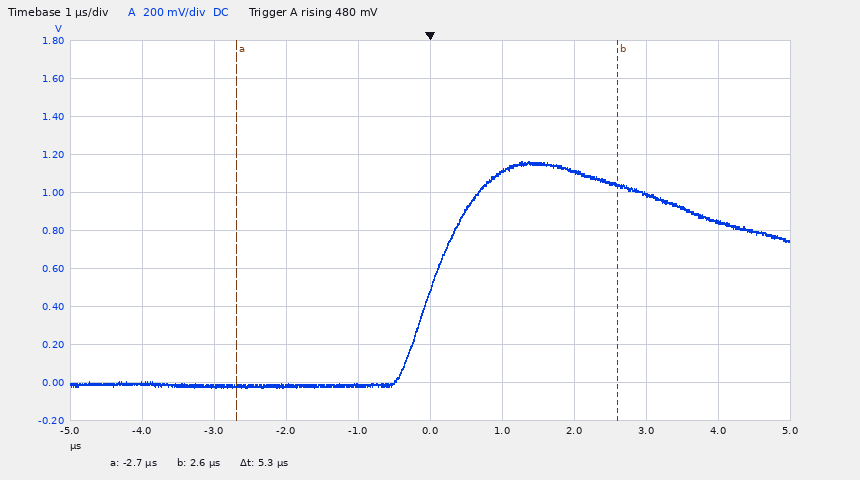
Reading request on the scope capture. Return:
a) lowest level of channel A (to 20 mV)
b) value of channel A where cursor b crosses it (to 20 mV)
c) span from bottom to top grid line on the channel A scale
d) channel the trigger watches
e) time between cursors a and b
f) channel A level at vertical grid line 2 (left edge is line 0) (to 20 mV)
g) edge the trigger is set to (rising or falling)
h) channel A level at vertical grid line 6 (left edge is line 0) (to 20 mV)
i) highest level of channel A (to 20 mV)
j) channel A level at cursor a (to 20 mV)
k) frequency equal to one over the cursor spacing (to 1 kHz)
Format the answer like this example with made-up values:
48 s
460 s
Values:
-20 mV
1.04 V
2 V
channel A
5.3 µs
-20 mV
rising
1.12 V
1.16 V
-20 mV
189 kHz
